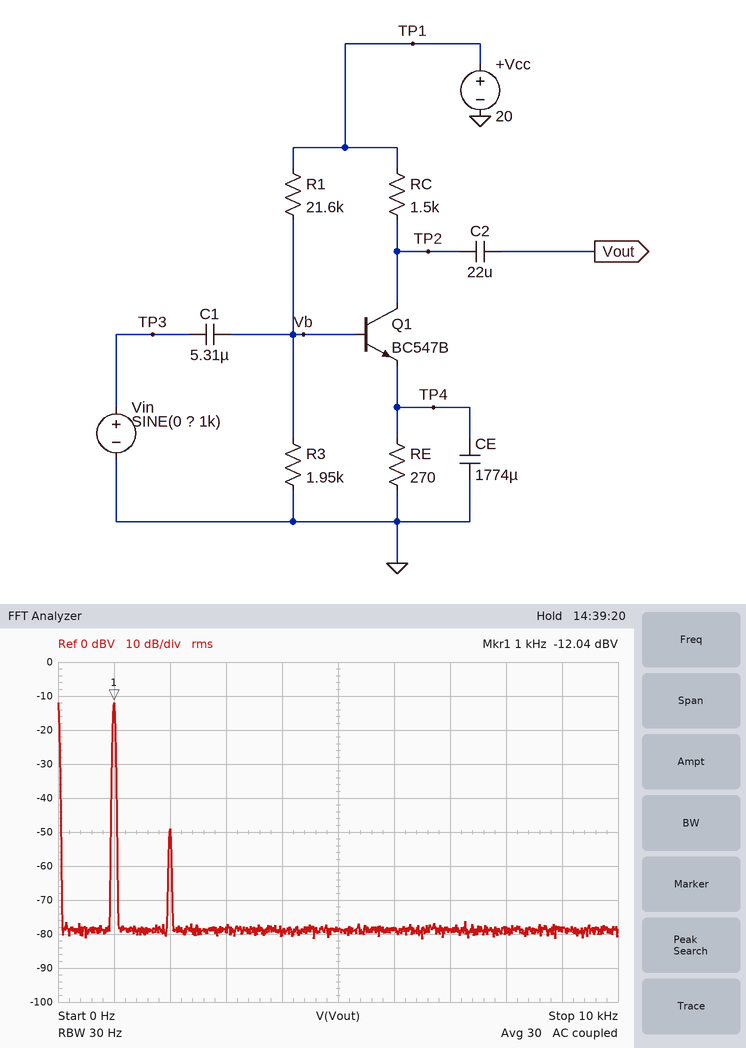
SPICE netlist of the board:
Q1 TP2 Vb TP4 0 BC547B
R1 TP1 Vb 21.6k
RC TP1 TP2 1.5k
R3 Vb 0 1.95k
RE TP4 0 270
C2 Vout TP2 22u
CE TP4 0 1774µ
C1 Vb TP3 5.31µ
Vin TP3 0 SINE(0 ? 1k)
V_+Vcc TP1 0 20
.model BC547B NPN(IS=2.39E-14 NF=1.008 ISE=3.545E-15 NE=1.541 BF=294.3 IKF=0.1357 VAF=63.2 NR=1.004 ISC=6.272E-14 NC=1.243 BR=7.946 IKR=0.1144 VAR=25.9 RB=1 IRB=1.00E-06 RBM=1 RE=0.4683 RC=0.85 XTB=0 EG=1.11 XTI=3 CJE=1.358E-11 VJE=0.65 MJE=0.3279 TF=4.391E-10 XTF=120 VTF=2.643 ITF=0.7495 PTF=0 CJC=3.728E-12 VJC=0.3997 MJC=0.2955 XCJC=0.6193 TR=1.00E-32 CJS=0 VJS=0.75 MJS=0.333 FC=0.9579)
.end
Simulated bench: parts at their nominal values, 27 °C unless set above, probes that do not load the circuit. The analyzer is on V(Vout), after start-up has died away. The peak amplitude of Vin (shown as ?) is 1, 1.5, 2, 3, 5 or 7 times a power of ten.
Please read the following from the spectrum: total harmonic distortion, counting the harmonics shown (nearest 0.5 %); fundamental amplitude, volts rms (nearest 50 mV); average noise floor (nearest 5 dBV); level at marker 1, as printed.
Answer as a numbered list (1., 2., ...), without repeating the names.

1. 1.5 %
2. 250 mV
3. -80 dBV
4. -12.04 dBV
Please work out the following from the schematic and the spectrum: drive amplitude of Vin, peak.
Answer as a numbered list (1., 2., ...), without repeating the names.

1. 2 mV
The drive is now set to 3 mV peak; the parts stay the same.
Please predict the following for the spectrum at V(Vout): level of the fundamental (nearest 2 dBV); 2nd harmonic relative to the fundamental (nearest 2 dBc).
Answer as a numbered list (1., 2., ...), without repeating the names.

1. -8 dBV
2. -34 dBc
